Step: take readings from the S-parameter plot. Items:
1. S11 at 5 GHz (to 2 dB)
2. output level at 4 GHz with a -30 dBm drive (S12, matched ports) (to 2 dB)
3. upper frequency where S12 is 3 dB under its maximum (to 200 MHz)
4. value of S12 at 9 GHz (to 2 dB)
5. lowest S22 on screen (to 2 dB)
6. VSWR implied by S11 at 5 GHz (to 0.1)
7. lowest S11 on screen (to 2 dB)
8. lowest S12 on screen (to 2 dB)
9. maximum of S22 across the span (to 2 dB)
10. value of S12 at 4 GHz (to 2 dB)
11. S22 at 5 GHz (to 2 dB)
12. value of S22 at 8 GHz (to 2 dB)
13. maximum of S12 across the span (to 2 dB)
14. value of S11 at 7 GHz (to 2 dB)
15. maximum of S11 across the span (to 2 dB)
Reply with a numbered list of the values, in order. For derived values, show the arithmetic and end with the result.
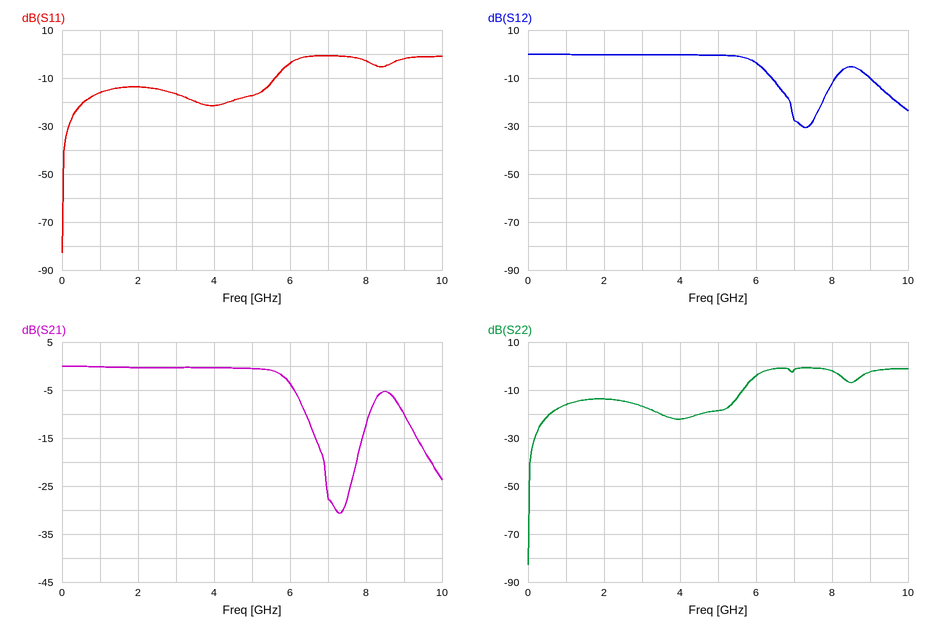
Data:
1. -18 dB
2. -30 dBm + (0 dB) = -30 dBm
3. 6.0 GHz
4. -10 dB
5. -82 dB
6. |Γ| = 10^(-18/20) = 0.1259; VSWR = (1 + 0.1259)/(1 − 0.1259) ≈ 1.3
7. -82 dB
8. -30 dB
9. 0 dB
10. 0 dB
11. -18 dB
12. -2 dB
13. 0 dB
14. 0 dB
15. 0 dB
